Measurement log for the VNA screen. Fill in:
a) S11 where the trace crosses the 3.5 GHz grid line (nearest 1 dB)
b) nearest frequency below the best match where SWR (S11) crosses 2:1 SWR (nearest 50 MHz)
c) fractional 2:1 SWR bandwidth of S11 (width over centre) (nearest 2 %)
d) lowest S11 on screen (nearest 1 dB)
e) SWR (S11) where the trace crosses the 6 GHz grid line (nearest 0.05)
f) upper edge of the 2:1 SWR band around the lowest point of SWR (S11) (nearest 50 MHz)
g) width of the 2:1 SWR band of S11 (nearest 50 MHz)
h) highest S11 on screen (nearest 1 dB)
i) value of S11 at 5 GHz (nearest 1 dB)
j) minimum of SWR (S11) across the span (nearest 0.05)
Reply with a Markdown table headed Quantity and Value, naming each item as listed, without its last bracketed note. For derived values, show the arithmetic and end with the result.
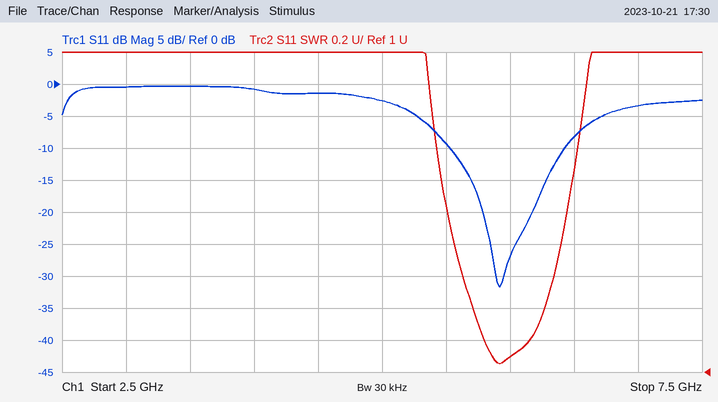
| Quantity | Value |
|---|---|
| S11 where the trace crosses the 3.5 GHz grid line | 0 dB |
| nearest frequency below the best match where SWR (S11) crosses 2:1 SWR | 5.50 GHz |
| fractional 2:1 SWR bandwidth of S11 (width over centre) | 950 MHz / 5.975 GHz ≈ 16 % |
| lowest S11 on screen | -32 dB |
| SWR (S11) where the trace crosses the 6 GHz grid line | 1.10 |
| upper edge of the 2:1 SWR band around the lowest point of SWR (S11) | 6.45 GHz |
| width of the 2:1 SWR band of S11 | 6.45 GHz − 5.50 GHz = 950 MHz |
| highest S11 on screen | 0 dB |
| value of S11 at 5 GHz | -3 dB |
| minimum of SWR (S11) across the span | 1.05 |
